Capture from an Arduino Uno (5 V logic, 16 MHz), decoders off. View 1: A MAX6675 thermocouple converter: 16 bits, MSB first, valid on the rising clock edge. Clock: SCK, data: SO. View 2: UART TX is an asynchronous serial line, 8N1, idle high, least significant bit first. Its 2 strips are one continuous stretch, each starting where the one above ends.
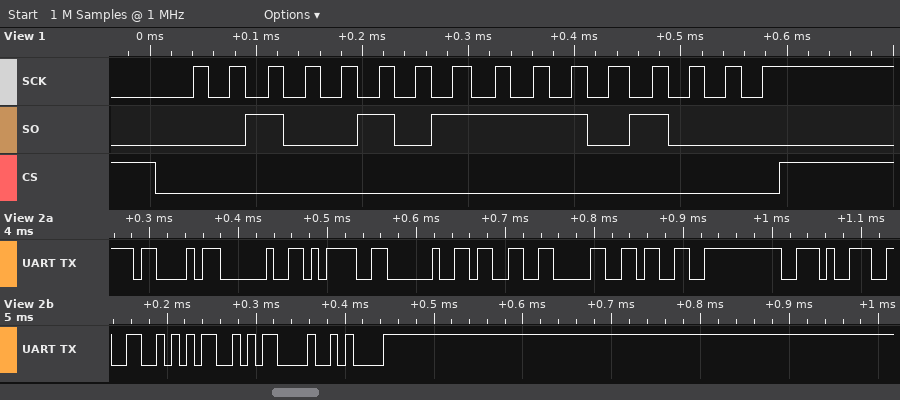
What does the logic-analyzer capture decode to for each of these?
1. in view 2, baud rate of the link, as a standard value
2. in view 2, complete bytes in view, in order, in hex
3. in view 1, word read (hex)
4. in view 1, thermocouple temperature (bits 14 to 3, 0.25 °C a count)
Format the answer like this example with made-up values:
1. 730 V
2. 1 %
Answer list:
1. 115200 baud
2. 43 20 3D 20 33 30 33 2E 32 35 0D 0A
3. 0x25E8
4. 303.25 °C
